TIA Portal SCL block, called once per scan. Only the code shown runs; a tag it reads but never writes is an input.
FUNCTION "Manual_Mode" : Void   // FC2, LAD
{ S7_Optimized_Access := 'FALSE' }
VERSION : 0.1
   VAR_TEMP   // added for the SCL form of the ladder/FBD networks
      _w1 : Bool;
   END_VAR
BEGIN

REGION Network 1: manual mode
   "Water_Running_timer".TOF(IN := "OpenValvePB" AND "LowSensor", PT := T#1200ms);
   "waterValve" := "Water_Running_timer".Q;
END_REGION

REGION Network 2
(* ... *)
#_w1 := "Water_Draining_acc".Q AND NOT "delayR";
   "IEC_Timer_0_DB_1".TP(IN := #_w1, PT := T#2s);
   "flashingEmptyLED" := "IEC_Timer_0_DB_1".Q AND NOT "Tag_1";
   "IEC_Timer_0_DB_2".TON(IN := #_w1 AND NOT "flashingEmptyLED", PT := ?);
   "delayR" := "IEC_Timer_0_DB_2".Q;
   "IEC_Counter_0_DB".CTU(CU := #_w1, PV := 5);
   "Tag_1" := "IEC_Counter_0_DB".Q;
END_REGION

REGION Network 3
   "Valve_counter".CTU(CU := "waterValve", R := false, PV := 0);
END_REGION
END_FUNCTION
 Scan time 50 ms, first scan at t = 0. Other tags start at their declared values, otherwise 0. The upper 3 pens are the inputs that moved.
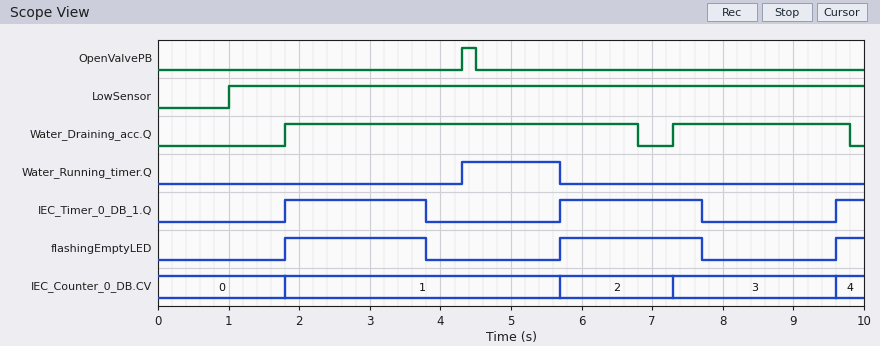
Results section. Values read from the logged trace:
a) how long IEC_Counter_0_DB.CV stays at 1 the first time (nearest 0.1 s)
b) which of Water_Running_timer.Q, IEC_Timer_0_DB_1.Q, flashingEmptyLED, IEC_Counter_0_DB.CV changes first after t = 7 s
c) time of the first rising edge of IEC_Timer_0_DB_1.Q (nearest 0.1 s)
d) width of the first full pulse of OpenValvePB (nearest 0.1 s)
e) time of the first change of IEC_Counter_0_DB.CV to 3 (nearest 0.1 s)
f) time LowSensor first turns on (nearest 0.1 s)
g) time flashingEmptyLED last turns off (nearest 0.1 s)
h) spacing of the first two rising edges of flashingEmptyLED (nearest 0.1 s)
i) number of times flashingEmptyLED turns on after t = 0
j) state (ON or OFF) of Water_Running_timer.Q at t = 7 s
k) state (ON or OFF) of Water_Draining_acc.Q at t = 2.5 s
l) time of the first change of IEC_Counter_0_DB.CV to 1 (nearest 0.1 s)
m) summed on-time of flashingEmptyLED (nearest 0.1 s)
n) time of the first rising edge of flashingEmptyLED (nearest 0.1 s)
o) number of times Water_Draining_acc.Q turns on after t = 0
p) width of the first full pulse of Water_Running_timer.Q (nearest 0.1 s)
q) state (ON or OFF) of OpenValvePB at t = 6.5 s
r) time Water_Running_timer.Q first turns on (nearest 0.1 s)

3.9 s
IEC_Counter_0_DB.CV
1.8 s
0.2 s
7.3 s
1.0 s
7.7 s
3.9 s
3
OFF
ON
1.8 s
4.4 s
1.8 s
2
1.4 s
OFF
4.3 s
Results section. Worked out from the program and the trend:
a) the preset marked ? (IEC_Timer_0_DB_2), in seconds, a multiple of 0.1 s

1.8 s
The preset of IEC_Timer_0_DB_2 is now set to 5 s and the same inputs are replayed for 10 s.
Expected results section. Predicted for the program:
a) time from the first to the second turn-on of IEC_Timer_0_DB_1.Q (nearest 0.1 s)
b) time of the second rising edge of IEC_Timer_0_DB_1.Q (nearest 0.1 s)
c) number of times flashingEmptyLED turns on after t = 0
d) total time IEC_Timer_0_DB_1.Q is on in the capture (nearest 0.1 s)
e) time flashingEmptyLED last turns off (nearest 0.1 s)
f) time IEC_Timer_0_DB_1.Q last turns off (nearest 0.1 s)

5.5 s
7.3 s
2
4.0 s
9.3 s
9.3 s
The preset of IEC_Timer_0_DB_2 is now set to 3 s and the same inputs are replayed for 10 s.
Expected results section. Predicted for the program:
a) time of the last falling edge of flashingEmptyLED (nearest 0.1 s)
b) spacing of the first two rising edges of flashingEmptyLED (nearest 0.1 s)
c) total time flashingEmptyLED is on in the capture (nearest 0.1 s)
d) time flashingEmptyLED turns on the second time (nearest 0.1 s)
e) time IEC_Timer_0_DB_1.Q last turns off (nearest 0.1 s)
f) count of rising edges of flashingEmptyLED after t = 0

9.3 s
5.5 s
4.0 s
7.3 s
9.3 s
2
